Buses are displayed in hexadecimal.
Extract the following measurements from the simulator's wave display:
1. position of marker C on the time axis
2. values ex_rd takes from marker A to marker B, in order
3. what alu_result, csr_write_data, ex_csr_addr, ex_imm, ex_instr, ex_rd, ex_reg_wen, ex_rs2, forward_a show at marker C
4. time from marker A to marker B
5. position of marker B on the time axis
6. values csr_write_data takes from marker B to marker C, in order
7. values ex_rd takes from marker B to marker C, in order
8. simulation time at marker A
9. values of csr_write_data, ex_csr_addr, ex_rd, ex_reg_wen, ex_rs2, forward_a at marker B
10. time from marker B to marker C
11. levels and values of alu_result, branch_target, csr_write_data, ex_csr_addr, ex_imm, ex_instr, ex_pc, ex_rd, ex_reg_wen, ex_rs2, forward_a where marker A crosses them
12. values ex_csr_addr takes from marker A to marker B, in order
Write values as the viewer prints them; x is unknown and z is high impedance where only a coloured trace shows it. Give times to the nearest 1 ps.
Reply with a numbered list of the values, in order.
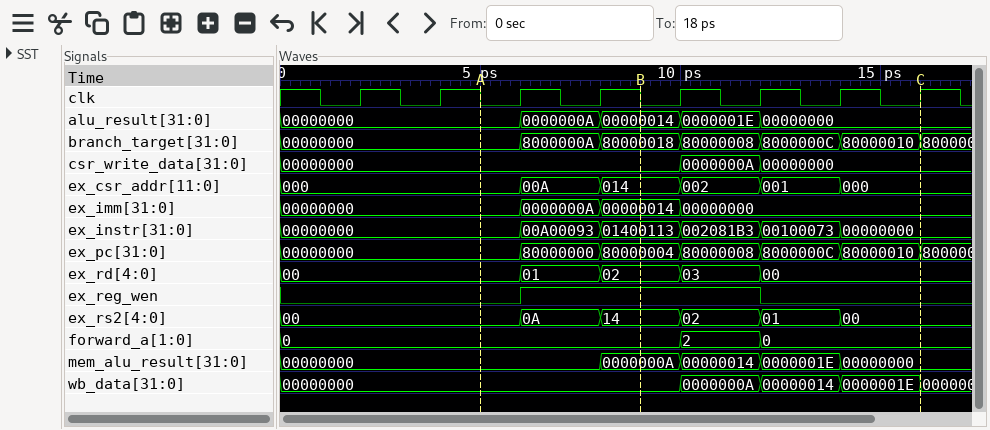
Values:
1. 16 ps
2. 00, 01, 02
3. alu_result=00000000, csr_write_data=00000000, ex_csr_addr=000, ex_imm=00000000, ex_instr=00000000, ex_rd=00, ex_reg_wen=0, ex_rs2=00, forward_a=0
4. 4 ps
5. 9 ps
6. 00000000, 0000000A, 00000000
7. 02, 03, 00
8. 5 ps
9. csr_write_data=00000000, ex_csr_addr=014, ex_rd=02, ex_reg_wen=1, ex_rs2=14, forward_a=0
10. 7 ps
11. alu_result=00000000, branch_target=00000000, csr_write_data=00000000, ex_csr_addr=000, ex_imm=00000000, ex_instr=00000000, ex_pc=00000000, ex_rd=00, ex_reg_wen=0, ex_rs2=00, forward_a=0
12. 000, 00A, 014
